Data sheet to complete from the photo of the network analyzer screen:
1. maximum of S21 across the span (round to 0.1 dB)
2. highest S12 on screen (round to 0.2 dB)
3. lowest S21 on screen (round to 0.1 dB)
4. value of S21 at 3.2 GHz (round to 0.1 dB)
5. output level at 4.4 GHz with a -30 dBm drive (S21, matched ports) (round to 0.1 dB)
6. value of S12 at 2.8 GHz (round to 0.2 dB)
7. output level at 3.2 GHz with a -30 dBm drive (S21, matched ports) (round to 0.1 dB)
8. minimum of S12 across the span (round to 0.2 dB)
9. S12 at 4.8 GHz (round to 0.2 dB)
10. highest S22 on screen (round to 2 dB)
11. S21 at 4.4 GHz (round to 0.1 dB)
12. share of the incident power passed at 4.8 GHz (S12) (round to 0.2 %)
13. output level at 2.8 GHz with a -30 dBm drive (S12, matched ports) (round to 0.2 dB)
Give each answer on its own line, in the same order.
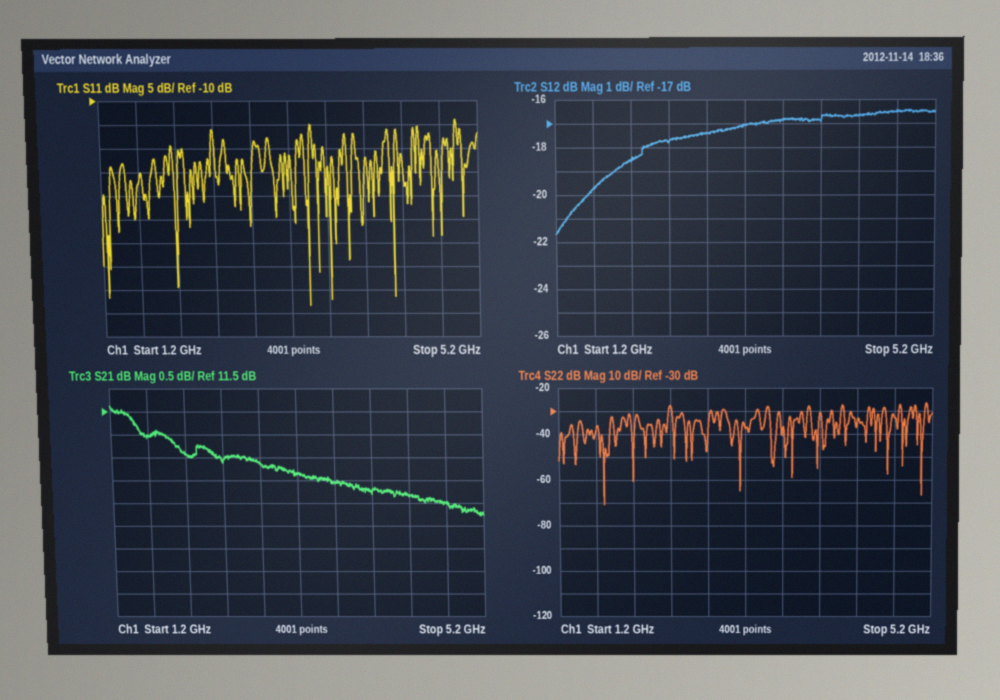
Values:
11.6 dB
-16.4 dB
9.2 dB
10.1 dB
-20.3 dBm
-17.4 dB
-19.9 dBm
-21.6 dB
-16.4 dB
-26 dB
9.7 dB
2.2 %
-47.4 dBm
